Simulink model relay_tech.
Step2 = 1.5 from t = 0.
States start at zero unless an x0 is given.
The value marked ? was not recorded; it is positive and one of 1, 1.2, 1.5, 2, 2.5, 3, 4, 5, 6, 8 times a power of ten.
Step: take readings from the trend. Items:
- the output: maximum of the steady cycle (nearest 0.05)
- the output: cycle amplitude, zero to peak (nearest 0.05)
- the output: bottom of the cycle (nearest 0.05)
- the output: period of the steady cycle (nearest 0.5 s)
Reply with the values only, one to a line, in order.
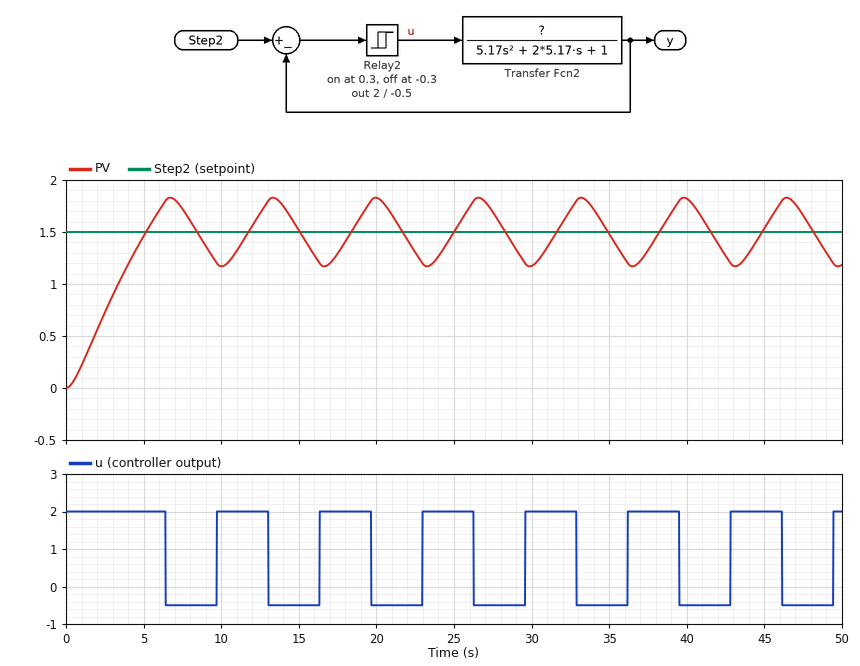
1.85
0.35
1.15
6.5 s
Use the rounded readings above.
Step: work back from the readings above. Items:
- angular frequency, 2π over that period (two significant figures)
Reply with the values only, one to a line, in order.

0.97 rad/s
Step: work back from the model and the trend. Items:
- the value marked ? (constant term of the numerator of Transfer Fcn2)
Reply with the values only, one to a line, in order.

2
